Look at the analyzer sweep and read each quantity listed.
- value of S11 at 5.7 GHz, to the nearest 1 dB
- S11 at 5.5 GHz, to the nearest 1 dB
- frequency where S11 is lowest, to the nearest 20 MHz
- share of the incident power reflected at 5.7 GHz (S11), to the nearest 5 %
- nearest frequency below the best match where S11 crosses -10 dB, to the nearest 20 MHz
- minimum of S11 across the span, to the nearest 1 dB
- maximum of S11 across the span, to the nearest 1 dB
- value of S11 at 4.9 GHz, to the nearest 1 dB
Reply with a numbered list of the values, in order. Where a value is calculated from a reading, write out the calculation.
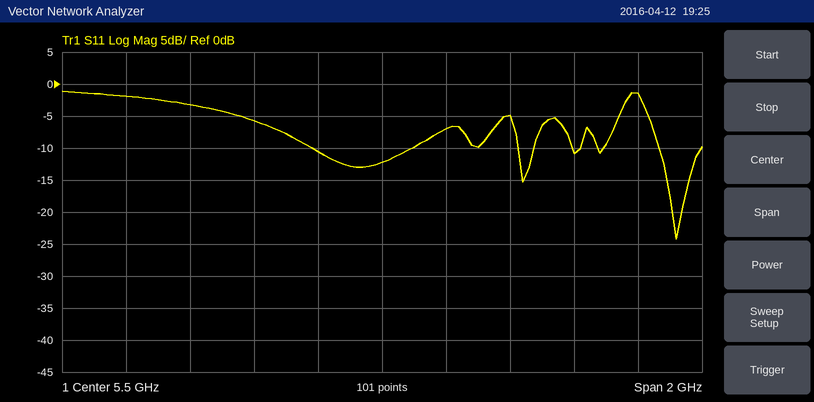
1. -7 dB
2. -12 dB
3. 6.42 GHz
4. 10^(-7/10) ≈ 20 %
5. 6.36 GHz
6. -24 dB
7. -1 dB
8. -3 dB
